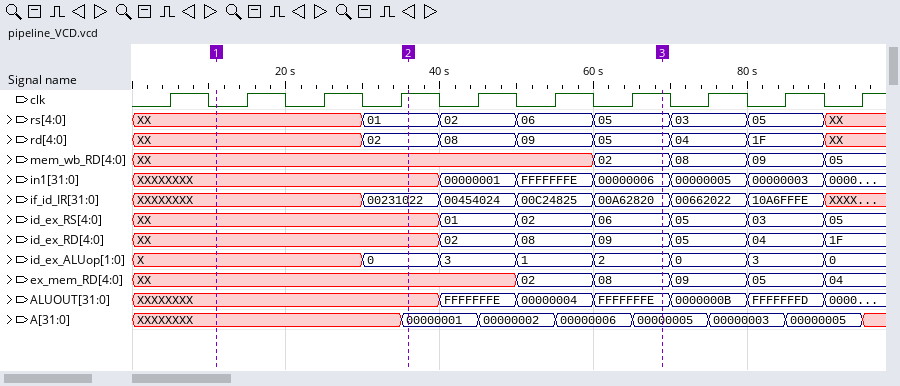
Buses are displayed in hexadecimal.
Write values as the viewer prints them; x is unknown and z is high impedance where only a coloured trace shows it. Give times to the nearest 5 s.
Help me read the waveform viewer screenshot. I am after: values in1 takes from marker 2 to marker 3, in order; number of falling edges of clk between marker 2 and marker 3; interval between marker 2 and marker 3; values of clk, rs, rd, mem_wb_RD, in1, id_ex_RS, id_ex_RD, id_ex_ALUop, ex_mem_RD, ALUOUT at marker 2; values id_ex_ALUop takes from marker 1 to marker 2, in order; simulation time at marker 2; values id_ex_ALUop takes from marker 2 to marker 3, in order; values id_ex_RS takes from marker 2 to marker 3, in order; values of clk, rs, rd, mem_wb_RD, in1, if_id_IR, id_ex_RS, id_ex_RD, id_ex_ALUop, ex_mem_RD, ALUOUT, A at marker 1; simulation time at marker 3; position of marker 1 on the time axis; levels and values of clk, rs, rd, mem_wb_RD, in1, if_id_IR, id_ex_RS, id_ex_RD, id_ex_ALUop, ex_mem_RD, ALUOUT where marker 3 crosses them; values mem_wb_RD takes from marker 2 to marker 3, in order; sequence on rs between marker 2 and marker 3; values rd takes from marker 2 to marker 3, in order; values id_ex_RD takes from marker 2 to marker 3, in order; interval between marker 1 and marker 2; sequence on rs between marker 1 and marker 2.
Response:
XXXXXXXX, 00000001, FFFFFFFE, 00000006
3
35 s
clk=1, rs=01, rd=02, mem_wb_RD=XX, in1=XXXXXXXX, id_ex_RS=XX, id_ex_RD=XX, id_ex_ALUop=0, ex_mem_RD=XX, ALUOUT=XXXXXXXX
X, 0
35 s
0, 3, 1, 2
XX, 01, 02, 06
clk=0, rs=XX, rd=XX, mem_wb_RD=XX, in1=XXXXXXXX, if_id_IR=XXXXXXXX, id_ex_RS=XX, id_ex_RD=XX, id_ex_ALUop=X, ex_mem_RD=XX, ALUOUT=XXXXXXXX, A=XXXXXXXX
70 s
10 s
clk=1, rs=05, rd=05, mem_wb_RD=02, in1=00000006, if_id_IR=00A62820, id_ex_RS=06, id_ex_RD=09, id_ex_ALUop=2, ex_mem_RD=08, ALUOUT=FFFFFFFE
XX, 02
01, 02, 06, 05
02, 08, 09, 05
XX, 02, 08, 09
25 s
XX, 01
